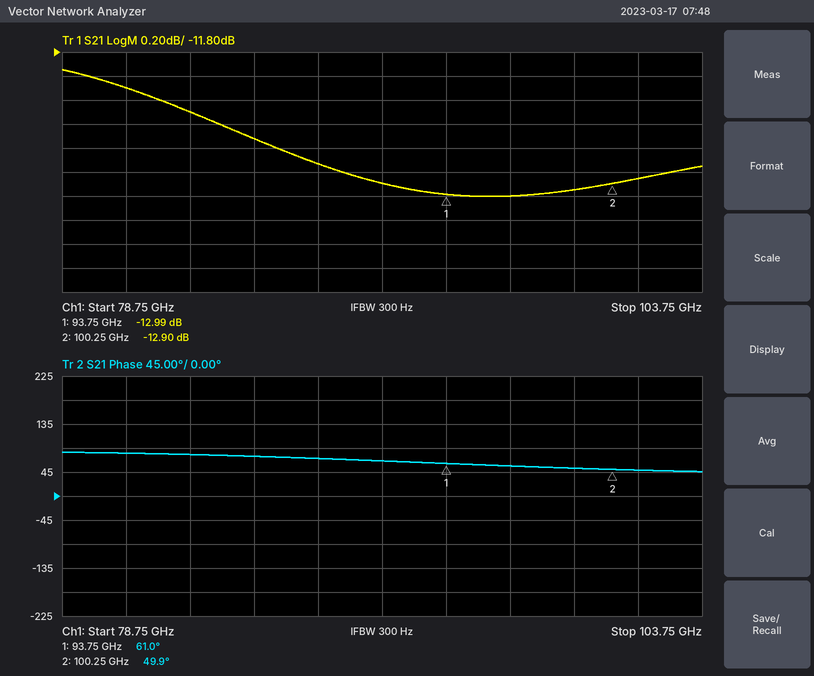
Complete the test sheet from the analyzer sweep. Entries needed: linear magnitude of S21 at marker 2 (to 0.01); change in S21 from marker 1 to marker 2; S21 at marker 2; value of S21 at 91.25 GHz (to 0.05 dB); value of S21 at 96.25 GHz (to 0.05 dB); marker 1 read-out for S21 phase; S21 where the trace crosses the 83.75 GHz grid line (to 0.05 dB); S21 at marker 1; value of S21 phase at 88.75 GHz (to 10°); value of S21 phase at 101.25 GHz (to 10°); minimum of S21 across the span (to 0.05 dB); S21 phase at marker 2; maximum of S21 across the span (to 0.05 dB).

0.23
0.09 dB
-12.90 dB
-12.90 dB
-13.00 dB
61.0°
-12.30 dB
-12.99 dB
70°
50°
-13.00 dB
49.9°
-11.95 dB
